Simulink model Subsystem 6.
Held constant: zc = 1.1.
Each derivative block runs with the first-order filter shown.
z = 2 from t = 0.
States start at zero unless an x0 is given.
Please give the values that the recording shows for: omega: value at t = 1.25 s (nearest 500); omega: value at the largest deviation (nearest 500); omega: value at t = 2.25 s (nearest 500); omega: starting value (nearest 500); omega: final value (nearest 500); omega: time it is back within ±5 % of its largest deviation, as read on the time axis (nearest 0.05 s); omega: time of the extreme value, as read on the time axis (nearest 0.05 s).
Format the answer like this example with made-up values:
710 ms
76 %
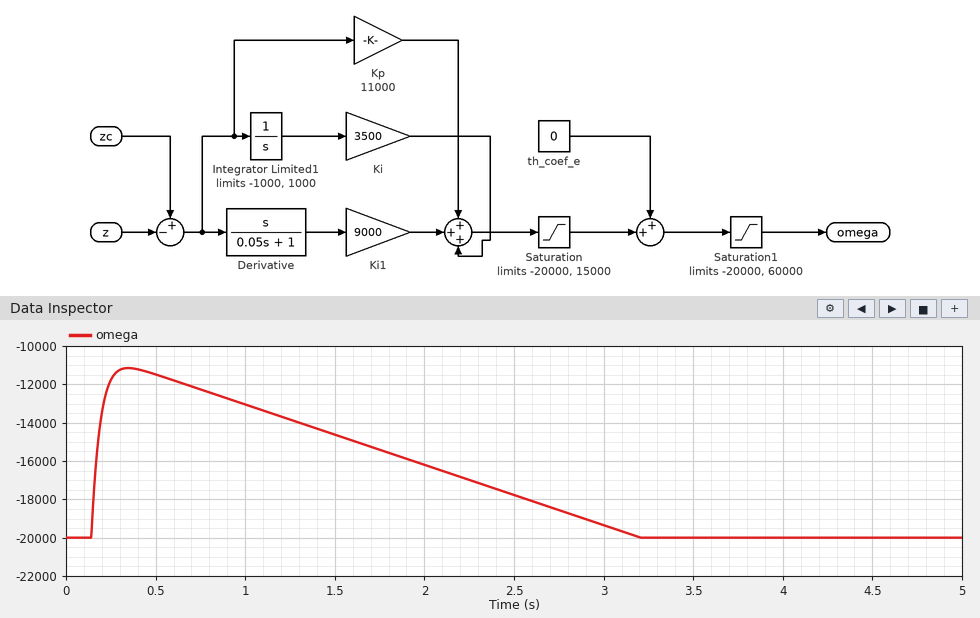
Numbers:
-14000
-11000
-17000
-20000
-20000
3.05 s
0.35 s
